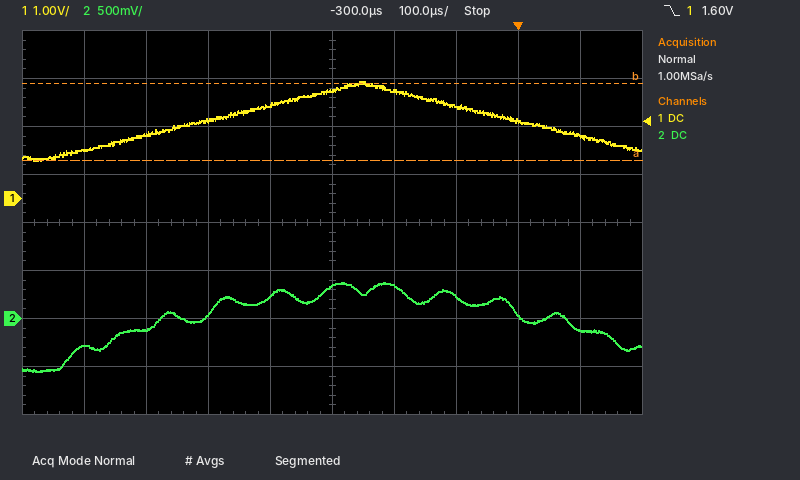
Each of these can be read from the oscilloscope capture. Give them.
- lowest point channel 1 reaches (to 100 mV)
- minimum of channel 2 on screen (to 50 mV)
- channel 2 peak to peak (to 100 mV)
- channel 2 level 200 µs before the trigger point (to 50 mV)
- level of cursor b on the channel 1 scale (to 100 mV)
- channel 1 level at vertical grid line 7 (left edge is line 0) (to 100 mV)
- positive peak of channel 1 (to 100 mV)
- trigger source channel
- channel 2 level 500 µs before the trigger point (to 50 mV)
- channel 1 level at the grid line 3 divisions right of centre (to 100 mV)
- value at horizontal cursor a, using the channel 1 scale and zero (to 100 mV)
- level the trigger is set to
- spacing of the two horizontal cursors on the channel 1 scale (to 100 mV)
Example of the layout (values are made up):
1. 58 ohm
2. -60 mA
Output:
1. 800 mV
2. -550 mV
3. 900 mV
4. 350 mV
5. 2.4 V
6. 1.9 V
7. 2.4 V
8. channel 1
9. 50 mV
10. 1.6 V
11. 800 mV
12. 1.60 V
13. 1.6 V
